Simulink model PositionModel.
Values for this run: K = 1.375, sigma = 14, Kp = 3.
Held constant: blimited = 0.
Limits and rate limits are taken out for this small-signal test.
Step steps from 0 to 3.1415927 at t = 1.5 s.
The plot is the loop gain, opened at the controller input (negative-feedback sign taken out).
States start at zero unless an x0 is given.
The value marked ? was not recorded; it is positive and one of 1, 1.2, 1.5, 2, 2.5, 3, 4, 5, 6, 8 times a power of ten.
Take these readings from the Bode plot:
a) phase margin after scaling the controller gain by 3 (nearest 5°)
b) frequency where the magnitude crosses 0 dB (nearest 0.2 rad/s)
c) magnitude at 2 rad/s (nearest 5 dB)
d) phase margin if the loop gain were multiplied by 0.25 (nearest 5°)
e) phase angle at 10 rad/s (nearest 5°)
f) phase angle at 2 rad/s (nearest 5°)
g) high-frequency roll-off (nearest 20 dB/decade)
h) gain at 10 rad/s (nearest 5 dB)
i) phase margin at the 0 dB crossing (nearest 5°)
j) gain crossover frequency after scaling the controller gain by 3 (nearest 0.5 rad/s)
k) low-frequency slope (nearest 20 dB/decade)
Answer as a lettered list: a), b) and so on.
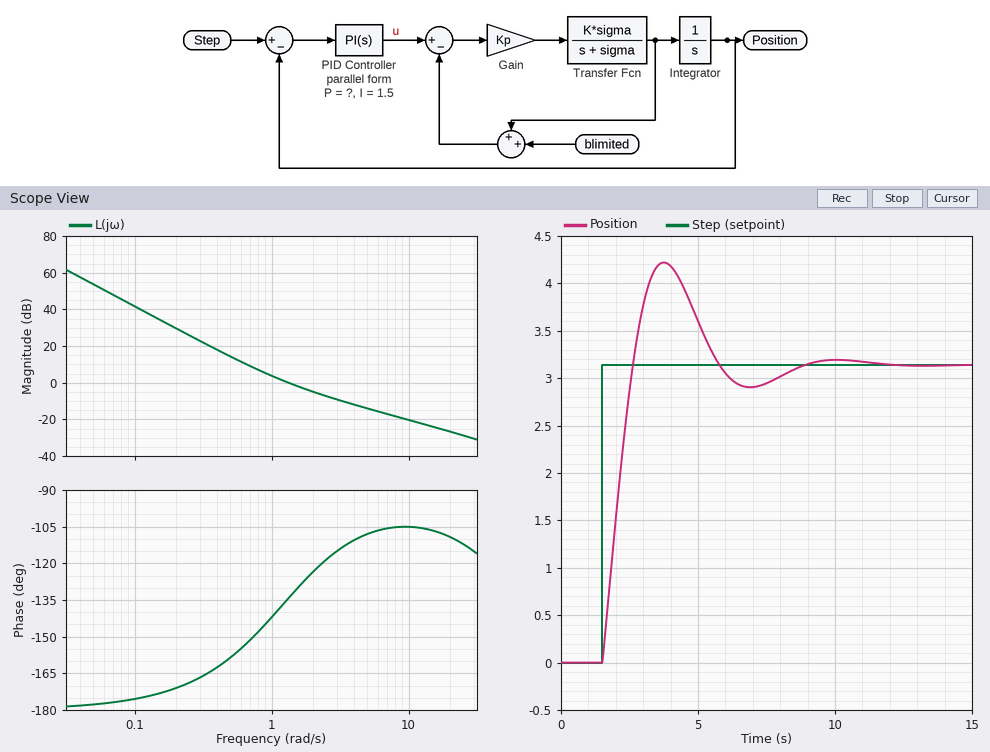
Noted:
a) 65°
b) 1.4 rad/s
c) -5 dB
d) 25°
e) -105°
f) -125°
g) -20 dB/decade
h) -20 dB
i) 45°
j) 3.0 rad/s
k) -40 dB/decade
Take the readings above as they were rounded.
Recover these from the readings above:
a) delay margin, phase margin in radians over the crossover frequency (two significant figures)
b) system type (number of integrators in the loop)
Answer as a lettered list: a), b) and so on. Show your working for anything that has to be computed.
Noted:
a) 45 × π / 180 / 1.4 = 0.56 s
b) 2
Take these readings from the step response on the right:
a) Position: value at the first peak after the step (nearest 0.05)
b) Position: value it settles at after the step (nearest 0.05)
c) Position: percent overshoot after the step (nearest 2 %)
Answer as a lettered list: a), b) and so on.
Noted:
a) 4.20
b) 3.15
c) 34 %
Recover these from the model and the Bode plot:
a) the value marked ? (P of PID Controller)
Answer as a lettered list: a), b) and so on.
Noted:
a) 1.2
